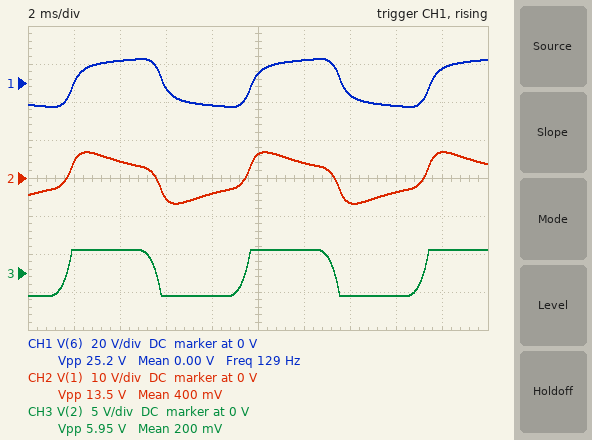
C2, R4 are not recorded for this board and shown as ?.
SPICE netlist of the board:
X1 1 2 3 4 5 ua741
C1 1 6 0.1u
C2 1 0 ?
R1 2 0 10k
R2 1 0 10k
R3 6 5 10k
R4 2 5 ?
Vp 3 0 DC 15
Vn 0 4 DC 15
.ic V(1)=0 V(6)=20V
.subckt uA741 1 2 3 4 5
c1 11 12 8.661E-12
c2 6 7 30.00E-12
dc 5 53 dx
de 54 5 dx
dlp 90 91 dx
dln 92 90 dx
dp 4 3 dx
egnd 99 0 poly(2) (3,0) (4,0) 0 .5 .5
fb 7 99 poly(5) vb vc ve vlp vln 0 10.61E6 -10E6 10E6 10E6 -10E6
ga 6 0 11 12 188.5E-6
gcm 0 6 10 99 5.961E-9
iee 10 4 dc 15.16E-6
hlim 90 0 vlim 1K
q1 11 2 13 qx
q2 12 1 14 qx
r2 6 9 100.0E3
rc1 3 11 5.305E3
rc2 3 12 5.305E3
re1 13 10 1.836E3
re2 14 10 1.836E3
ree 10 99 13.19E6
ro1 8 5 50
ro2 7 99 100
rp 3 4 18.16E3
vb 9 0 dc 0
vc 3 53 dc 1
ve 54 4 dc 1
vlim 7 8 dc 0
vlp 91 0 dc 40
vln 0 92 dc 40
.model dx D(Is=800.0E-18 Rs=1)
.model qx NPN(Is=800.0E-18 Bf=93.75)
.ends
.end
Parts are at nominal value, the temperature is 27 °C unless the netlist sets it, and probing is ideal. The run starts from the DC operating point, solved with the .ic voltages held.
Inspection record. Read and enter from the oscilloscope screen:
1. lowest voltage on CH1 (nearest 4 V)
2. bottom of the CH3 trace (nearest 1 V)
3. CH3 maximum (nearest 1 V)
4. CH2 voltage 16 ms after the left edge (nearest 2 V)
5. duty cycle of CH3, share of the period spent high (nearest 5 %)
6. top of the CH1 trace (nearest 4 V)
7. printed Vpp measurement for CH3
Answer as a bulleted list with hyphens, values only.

- -12 V
- -3 V
- 3 V
- -4 V
- 50 %
- 12 V
- 5.95 V
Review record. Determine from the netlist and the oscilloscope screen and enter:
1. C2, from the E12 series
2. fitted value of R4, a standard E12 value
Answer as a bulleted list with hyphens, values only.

- 82 nF
- 39 kΩ
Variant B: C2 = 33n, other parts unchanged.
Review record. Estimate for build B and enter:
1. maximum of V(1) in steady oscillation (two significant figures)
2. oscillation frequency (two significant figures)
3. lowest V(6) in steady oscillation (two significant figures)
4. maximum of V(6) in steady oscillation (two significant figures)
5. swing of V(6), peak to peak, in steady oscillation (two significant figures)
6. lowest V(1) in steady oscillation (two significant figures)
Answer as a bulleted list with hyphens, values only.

- 8.8 V
- 150 Hz
- -12 V
- 12 V
- 24 V
- -8.8 V
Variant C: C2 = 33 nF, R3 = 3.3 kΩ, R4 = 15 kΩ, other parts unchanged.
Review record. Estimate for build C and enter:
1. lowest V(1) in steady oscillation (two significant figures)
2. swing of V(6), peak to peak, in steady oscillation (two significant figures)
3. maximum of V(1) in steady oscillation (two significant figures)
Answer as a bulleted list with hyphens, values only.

- -11 V
- 26 V
- 11 V
